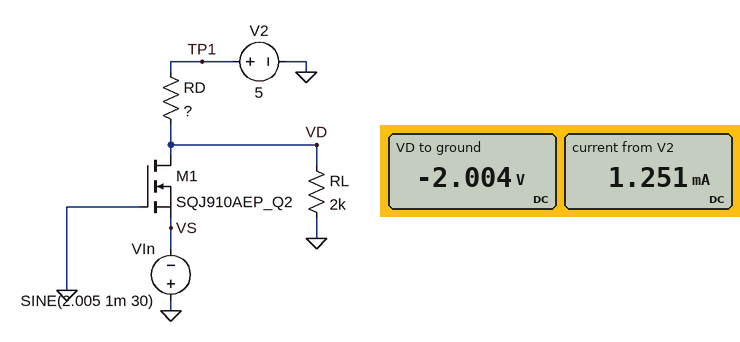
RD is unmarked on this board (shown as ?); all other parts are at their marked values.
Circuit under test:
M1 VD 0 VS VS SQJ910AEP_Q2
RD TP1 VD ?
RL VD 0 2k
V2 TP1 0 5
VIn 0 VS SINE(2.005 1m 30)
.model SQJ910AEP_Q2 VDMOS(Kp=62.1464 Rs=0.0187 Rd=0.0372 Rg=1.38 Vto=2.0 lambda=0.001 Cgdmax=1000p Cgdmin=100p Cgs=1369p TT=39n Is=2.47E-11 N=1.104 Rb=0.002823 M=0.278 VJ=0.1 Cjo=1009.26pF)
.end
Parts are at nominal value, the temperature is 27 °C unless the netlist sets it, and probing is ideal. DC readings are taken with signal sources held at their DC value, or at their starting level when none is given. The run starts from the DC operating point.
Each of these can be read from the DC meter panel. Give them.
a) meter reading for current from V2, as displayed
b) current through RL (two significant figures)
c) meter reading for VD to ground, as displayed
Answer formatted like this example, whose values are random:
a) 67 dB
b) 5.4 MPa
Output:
a) 1.251 mA
b) 1.0 mA
c) -2.004 V
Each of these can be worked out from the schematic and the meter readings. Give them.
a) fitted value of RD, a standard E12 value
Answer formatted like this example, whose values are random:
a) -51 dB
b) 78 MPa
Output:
a) 5.6 kΩ
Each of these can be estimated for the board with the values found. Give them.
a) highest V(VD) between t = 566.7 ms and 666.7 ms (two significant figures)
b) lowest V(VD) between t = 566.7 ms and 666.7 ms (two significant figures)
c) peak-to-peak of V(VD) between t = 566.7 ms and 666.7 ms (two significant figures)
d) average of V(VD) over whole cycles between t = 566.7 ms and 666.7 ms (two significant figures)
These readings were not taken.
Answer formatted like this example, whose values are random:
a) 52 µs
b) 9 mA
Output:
a) -2.0 V
b) -2.0 V
c) 2.0 mV
d) -2.0 V
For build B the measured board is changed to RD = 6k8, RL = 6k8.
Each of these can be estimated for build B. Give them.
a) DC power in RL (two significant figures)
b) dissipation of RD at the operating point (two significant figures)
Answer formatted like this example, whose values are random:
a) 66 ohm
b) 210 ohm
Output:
a) 590 µW
b) 7.2 mW
